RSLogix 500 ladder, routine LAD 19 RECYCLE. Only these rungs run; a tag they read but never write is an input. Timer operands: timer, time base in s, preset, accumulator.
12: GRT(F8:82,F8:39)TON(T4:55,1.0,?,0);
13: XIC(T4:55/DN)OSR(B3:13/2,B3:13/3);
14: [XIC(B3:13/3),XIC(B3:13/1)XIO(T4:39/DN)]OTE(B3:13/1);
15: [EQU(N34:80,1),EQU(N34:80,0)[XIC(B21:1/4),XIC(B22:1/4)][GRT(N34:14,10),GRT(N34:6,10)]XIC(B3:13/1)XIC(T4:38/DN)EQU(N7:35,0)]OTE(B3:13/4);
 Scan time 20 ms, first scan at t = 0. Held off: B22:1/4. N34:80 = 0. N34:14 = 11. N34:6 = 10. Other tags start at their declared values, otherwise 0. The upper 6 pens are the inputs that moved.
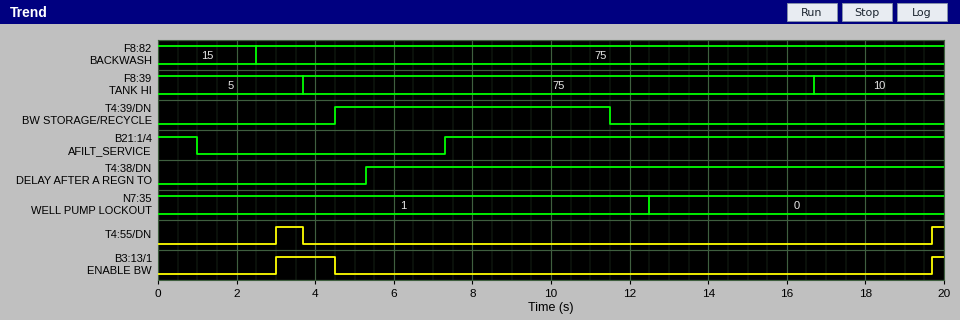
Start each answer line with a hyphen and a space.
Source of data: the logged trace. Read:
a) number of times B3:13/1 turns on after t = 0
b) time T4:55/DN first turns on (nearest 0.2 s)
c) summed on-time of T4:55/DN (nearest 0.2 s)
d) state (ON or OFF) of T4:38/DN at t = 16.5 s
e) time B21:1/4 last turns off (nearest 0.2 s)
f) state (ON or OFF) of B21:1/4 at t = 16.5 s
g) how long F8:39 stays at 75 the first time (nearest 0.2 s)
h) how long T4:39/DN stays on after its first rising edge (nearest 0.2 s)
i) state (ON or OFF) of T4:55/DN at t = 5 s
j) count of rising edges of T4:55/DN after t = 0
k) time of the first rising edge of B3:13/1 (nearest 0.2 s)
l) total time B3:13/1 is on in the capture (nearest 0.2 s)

- 2
- 3.0 s
- 1.0 s
- ON
- 1.0 s
- ON
- 13.0 s
- 7.0 s
- OFF
- 2
- 3.0 s
- 1.8 s
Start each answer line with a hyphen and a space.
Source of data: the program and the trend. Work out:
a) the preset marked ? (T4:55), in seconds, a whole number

- 3 s
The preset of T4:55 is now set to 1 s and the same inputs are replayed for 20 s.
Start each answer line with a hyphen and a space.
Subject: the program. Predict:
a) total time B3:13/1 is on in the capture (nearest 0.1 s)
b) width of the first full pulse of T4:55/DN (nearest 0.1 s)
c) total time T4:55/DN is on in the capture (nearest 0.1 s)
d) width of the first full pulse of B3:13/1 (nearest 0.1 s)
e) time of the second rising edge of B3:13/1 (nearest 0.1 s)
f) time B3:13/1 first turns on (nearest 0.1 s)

- 5.8 s
- 2.7 s
- 5.0 s
- 3.5 s
- 17.7 s
- 1.0 s
